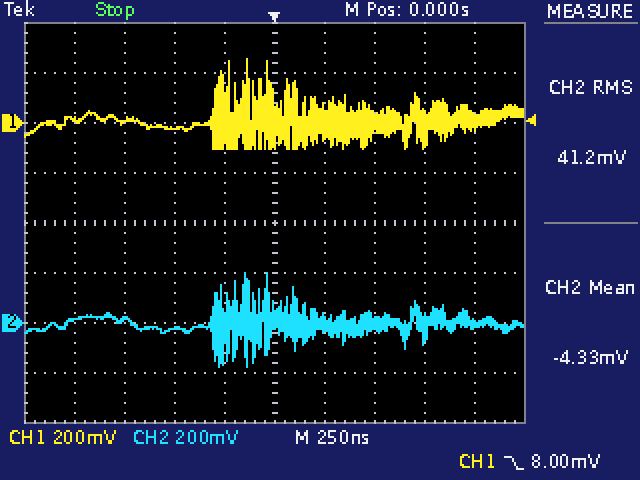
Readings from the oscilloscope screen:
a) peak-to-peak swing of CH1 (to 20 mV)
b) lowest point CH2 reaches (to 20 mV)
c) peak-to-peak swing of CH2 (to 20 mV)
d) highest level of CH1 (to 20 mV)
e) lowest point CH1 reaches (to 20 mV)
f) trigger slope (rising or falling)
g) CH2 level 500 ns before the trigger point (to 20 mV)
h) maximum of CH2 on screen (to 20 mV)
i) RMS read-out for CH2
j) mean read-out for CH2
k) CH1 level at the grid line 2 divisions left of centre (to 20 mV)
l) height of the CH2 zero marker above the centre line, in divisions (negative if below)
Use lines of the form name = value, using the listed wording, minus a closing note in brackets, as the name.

peak-to-peak swing of CH1 = 360 mV
lowest point CH2 reaches = -180 mV
peak-to-peak swing of CH2 = 380 mV
highest level of CH1 = 260 mV
lowest point CH1 reaches = -100 mV
trigger slope = falling
CH2 level 500 ns before the trigger point = -20 mV
maximum of CH2 on screen = 200 mV
RMS read-out for CH2 = 41.2 mV
mean read-out for CH2 = -4.33 mV
CH1 level at the grid line 2 divisions left of centre = -20 mV
height of the CH2 zero marker above the centre line, in divisions = -2.0 div
